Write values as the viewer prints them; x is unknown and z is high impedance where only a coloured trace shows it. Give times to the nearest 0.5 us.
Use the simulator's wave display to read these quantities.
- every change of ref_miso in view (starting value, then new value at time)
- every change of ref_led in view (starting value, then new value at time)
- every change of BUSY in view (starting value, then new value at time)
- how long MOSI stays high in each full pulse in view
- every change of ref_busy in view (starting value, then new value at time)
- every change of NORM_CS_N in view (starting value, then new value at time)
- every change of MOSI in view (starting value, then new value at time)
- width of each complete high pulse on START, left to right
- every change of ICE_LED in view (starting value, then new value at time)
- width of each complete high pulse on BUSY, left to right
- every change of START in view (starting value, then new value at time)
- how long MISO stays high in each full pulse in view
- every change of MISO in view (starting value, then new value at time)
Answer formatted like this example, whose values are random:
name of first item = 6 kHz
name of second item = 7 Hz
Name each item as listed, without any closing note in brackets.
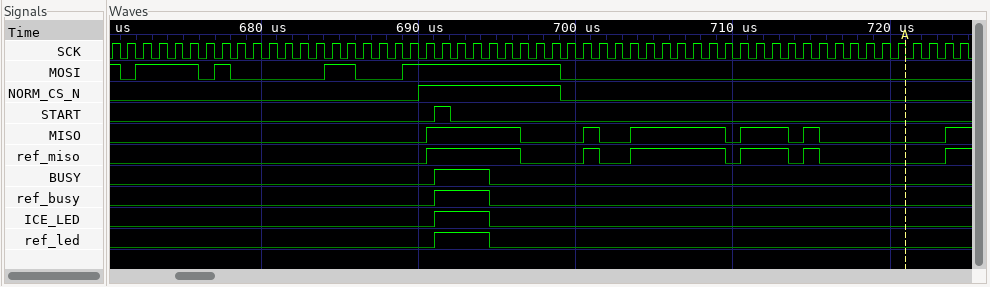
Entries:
every change of ref_miso in view = 0, 1 at 690.5 us, 0 at 696.5 us, 1 at 700.5 us, 0 at 701.5 us, 1 at 703.5 us, 0 at 709.5 us, 1 at 710.5 us, 0 at 713.5 us, 1 at 714.5 us, 0 at 715.5 us, 1 at 723.5 us
every change of ref_led in view = 0, 1 at 691 us, 0 at 694.5 us
every change of BUSY in view = 0, 1 at 691 us, 0 at 694.5 us
how long MOSI stays high in each full pulse in view = 4 us, 1 us, 2 us, 10 us
every change of ref_busy in view = 0, 1 at 691 us, 0 at 694.5 us
every change of NORM_CS_N in view = 0, 1 at 690 us, 0 at 699 us
every change of MOSI in view = 1, 0 at 671 us, 1 at 672 us, 0 at 676 us, 1 at 677 us, 0 at 678 us, 1 at 684 us, 0 at 686 us, 1 at 689 us, 0 at 699 us
width of each complete high pulse on START, left to right = 1 us
every change of ICE_LED in view = 0, 1 at 691 us, 0 at 694.5 us
width of each complete high pulse on BUSY, left to right = 3.5 us
every change of START in view = 0, 1 at 691 us, 0 at 692 us
how long MISO stays high in each full pulse in view = 6 us, 1 us, 6 us, 3 us, 1 us
every change of MISO in view = 0, 1 at 690.5 us, 0 at 696.5 us, 1 at 700.5 us, 0 at 701.5 us, 1 at 703.5 us, 0 at 709.5 us, 1 at 710.5 us, 0 at 713.5 us, 1 at 714.5 us, 0 at 715.5 us, 1 at 723.5 us
